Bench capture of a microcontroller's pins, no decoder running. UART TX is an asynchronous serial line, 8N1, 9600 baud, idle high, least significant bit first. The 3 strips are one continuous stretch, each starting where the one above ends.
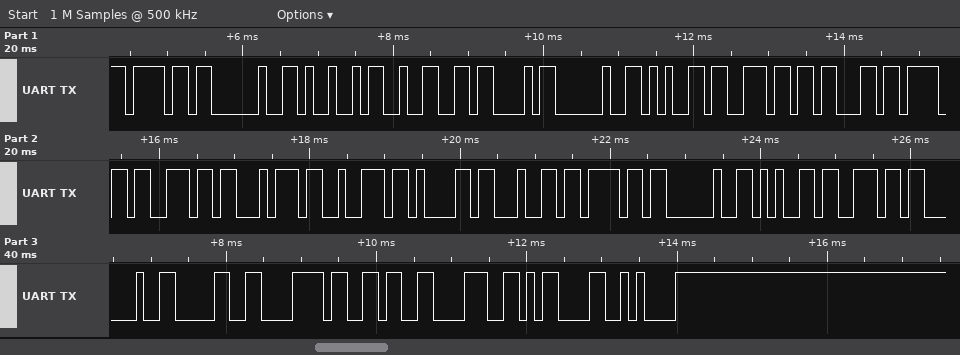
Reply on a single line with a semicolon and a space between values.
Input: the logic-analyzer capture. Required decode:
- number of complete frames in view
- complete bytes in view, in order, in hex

26; 0x6F 0x20 0x49 0x32 0x43 0x20 0x65 0x6E 0x63 0x6F 0x6E 0x74 0x72 0x61 0x64 0x6F 0x20 0x65 0x6E 0x20 0x30 0x78 0x36 0x38 0x0D 0x0A
